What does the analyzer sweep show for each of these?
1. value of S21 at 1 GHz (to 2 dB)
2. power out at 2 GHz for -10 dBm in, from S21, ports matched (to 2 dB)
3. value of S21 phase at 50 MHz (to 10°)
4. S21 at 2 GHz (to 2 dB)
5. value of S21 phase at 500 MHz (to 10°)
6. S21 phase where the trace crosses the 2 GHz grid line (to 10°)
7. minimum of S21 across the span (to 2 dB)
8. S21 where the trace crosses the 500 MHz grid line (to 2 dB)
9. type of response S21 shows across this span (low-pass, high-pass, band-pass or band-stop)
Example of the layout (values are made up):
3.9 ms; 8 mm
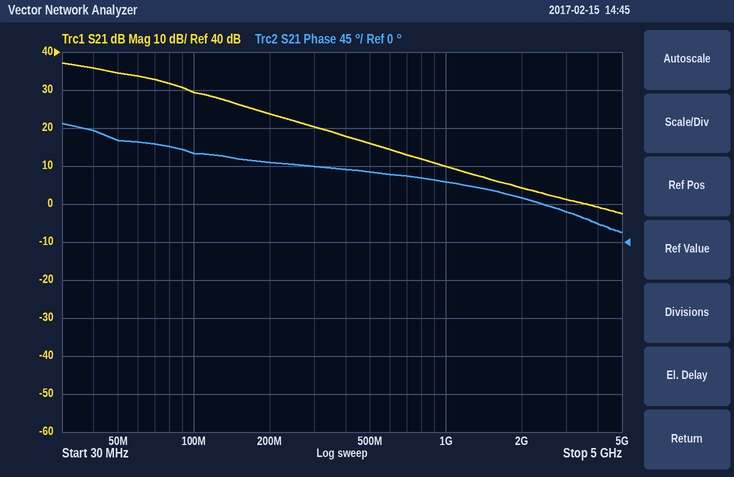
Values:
10 dB; -6 dBm; 120°; 4 dB; 80°; 50°; -2 dB; 16 dB; low-pass
